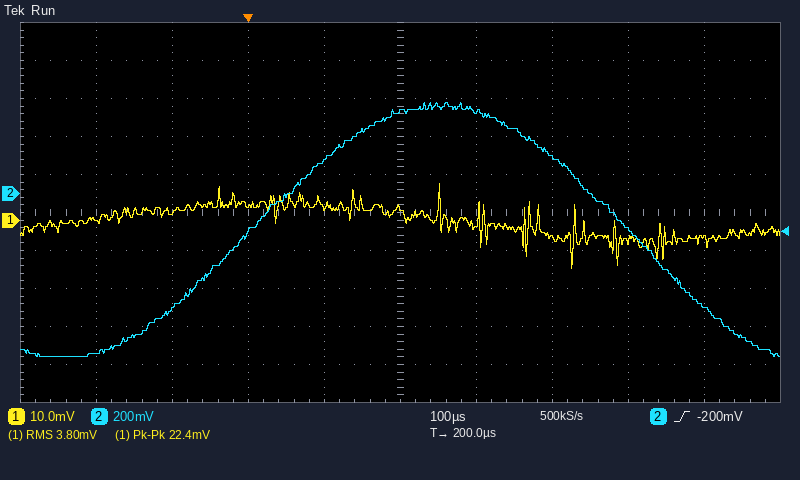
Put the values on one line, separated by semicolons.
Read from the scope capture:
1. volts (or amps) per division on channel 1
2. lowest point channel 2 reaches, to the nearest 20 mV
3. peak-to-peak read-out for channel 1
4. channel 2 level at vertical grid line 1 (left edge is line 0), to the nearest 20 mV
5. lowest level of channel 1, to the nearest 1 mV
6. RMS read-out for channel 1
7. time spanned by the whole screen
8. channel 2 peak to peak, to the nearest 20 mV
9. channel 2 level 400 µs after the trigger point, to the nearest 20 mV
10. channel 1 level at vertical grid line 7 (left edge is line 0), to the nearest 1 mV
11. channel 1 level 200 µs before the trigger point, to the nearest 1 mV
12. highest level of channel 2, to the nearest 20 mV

10 mV; -860 mV; 22.4 mV; -840 mV; -13 mV; 3.80 mV; 1 ms; 1.34 V; 200 mV; -5 mV; 0 mV; 480 mV
